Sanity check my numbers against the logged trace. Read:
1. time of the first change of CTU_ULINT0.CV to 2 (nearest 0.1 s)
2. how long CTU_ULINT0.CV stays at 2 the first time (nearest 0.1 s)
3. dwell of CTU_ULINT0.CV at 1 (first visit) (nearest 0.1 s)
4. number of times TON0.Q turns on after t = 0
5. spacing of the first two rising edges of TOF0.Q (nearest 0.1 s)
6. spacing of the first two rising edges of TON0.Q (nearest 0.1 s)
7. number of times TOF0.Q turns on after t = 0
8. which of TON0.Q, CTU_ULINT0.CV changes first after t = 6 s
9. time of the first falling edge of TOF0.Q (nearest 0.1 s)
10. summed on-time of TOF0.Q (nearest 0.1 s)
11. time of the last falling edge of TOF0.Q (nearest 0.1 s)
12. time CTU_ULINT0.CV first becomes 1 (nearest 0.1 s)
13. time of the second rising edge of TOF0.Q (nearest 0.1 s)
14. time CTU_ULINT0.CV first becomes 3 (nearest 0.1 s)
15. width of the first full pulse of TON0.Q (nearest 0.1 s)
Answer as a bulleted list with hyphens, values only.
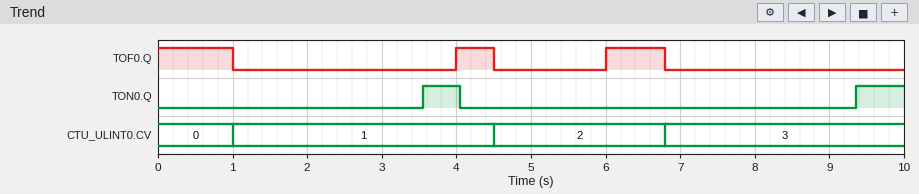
- 4.5 s
- 2.3 s
- 3.5 s
- 2
- 2.0 s
- 5.8 s
- 2
- CTU_ULINT0.CV
- 1.0 s
- 2.3 s
- 6.8 s
- 1.0 s
- 6.0 s
- 6.8 s
- 0.5 s
